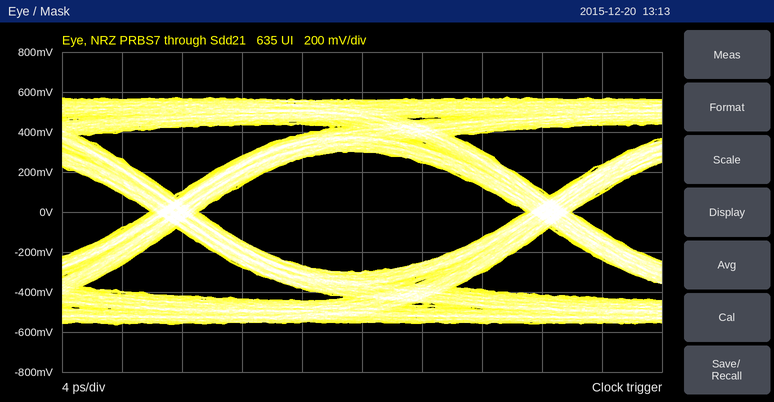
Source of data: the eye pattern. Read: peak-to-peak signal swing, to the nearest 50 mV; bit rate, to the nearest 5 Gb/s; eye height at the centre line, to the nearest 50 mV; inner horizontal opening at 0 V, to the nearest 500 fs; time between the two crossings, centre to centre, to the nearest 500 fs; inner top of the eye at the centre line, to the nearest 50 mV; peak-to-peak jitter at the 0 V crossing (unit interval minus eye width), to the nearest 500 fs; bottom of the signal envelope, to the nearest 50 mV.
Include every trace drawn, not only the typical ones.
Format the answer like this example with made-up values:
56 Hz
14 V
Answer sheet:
1.15 V
40 Gb/s
600 mV
22.0 ps
25.0 ps
300 mV
3.0 ps
-550 mV
